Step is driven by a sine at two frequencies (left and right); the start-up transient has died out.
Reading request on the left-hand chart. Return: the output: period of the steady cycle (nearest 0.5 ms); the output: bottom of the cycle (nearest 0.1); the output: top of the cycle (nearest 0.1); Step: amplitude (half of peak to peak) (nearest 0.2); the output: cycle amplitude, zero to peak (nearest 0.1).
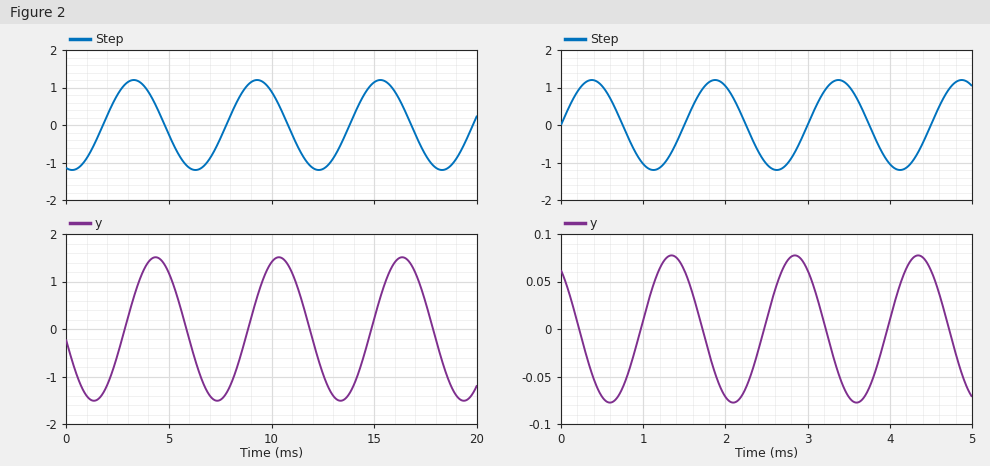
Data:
6.0 ms
-1.5
1.5
1.2
1.5
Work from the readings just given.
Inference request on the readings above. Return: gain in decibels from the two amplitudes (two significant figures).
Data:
1.9 dB
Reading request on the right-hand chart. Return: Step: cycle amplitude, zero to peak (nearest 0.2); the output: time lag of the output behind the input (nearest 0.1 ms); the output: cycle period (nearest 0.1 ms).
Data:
1.2
1.0 ms
1.5 ms
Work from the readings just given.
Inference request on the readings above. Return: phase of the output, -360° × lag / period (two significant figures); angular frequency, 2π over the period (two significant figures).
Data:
-240°
4.2 rad/ms
